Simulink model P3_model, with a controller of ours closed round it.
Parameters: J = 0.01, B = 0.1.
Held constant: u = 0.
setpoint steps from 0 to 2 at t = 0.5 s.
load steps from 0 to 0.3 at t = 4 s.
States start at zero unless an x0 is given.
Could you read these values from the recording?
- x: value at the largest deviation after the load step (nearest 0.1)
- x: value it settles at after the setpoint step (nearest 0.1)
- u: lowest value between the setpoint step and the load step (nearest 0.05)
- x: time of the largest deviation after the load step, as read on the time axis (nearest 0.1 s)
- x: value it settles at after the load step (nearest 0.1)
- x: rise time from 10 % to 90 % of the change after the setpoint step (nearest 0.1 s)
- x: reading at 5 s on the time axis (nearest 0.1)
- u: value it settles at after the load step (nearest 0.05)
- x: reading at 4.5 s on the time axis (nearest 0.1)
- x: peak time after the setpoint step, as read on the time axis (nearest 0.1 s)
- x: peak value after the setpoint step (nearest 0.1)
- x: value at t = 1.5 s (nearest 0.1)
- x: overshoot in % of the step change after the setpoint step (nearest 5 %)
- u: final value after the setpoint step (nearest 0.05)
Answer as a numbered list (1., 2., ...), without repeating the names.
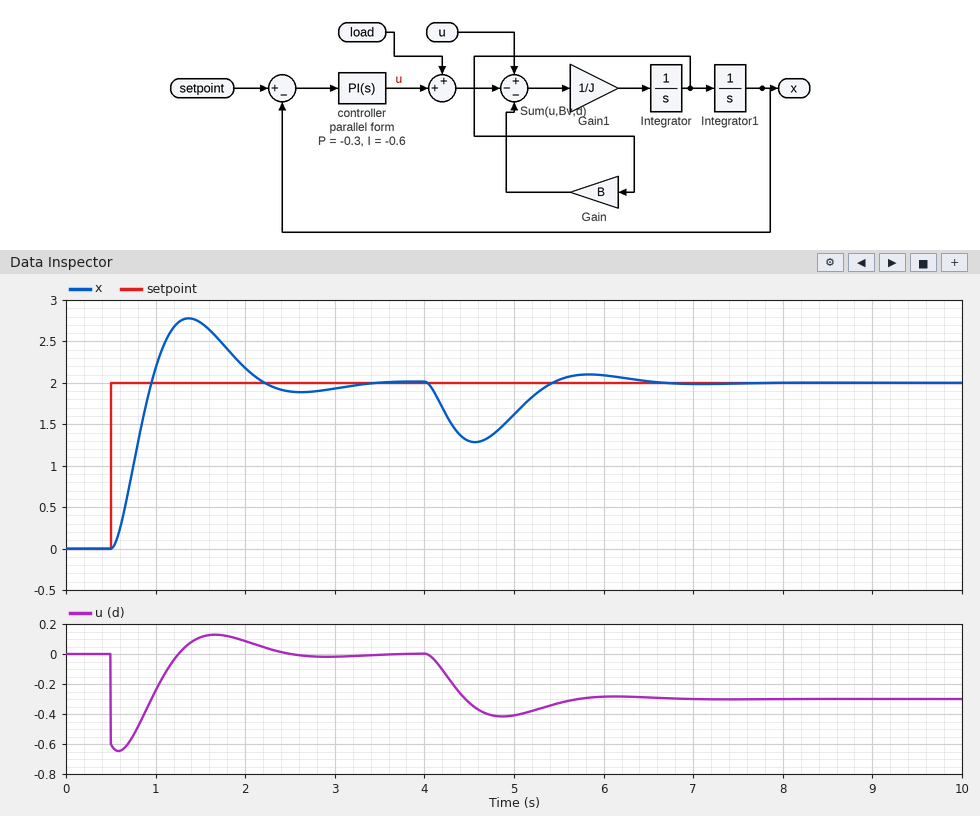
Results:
1. 1.3
2. 2.0
3. -0.65
4. 4.6 s
5. 2.0
6. 0.3 s
7. 1.6
8. -0.30
9. 1.3
10. 1.4 s
11. 2.8
12. 2.7
13. 40 %
14. 0.00
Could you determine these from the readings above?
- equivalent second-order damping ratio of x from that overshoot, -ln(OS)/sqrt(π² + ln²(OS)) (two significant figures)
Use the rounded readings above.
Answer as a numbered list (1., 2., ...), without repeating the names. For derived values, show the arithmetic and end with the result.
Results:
1. ln(0.4) = -0.916; 0.916 / sqrt(9.870 + 0.840) = 0.28
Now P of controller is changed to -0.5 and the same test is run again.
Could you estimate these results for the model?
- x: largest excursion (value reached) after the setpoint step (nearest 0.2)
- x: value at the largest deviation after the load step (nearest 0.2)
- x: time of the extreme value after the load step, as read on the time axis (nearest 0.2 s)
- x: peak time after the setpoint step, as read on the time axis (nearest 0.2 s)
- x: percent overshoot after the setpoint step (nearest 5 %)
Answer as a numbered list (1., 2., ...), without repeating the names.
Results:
1. 2.6
2. 1.4
3. 4.4 s
4. 1.2 s
5. 25 %
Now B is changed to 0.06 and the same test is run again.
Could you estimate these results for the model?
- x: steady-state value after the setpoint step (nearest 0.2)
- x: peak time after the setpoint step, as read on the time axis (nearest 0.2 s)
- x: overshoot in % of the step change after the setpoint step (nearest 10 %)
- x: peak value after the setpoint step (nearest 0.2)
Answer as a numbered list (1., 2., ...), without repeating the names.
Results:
1. 2.0
2. 1.2 s
3. 50 %
4. 3.0
